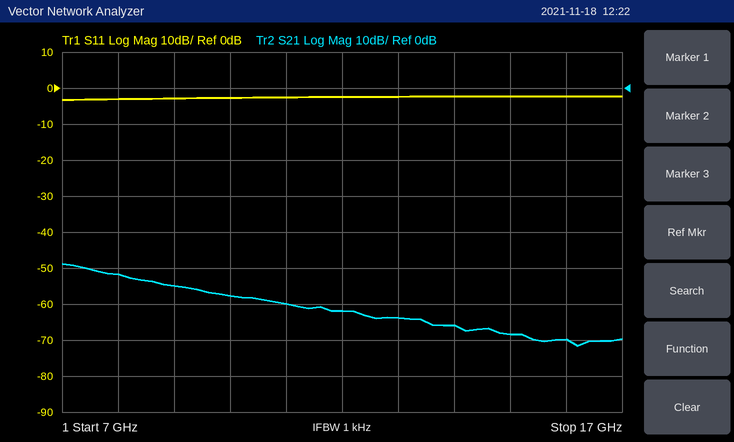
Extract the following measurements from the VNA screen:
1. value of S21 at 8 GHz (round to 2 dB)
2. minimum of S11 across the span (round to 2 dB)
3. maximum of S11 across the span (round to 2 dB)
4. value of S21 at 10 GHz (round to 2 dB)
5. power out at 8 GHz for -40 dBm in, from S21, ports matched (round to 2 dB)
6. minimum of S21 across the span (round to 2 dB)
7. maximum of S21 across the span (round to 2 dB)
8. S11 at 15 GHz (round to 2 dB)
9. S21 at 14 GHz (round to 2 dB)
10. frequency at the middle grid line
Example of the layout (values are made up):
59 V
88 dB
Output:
-52 dB
-4 dB
-2 dB
-58 dB
-92 dBm
-72 dB
-48 dB
-2 dB
-66 dB
12 GHz
